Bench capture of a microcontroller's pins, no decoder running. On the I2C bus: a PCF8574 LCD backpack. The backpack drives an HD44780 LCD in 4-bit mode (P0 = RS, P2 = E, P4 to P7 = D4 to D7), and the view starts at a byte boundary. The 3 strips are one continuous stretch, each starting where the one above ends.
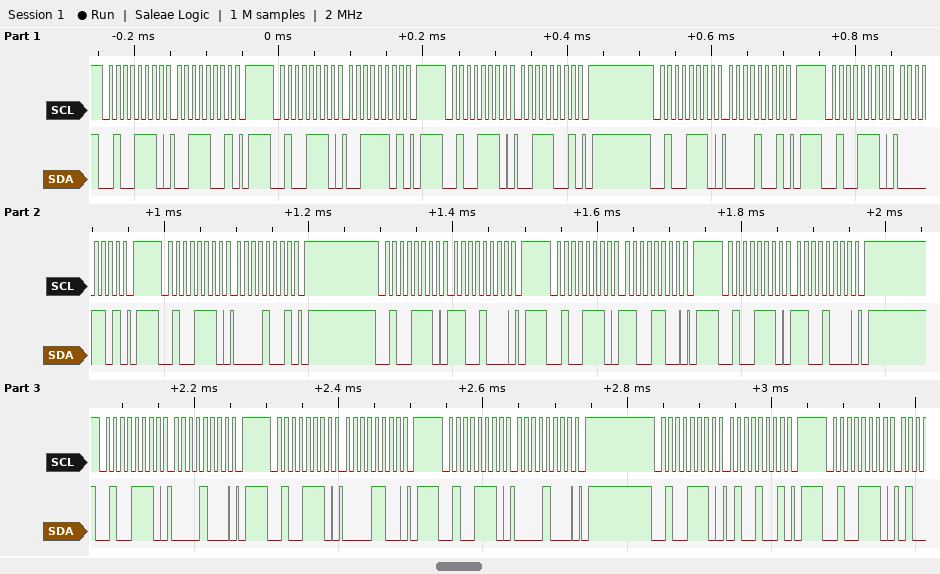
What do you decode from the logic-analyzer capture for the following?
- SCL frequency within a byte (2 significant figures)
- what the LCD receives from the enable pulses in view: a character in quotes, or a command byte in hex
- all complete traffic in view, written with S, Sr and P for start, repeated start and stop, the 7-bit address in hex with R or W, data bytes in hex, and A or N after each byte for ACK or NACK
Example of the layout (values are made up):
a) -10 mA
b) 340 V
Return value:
a) 100 kHz
b) '0' 0xC0
c) S 27W A 39 A P S 27W A 3D A P S 27W A 39 A P S 27W A 09 A P S 27W A 0D A P S 27W A 09 A P S 27W A C8 A P S 27W A CC A P S 27W A C8 A P S 27W A 08 A P S 27W A 0C A P S 27W A 08 A P S 27W A 49 A P S 27W A
